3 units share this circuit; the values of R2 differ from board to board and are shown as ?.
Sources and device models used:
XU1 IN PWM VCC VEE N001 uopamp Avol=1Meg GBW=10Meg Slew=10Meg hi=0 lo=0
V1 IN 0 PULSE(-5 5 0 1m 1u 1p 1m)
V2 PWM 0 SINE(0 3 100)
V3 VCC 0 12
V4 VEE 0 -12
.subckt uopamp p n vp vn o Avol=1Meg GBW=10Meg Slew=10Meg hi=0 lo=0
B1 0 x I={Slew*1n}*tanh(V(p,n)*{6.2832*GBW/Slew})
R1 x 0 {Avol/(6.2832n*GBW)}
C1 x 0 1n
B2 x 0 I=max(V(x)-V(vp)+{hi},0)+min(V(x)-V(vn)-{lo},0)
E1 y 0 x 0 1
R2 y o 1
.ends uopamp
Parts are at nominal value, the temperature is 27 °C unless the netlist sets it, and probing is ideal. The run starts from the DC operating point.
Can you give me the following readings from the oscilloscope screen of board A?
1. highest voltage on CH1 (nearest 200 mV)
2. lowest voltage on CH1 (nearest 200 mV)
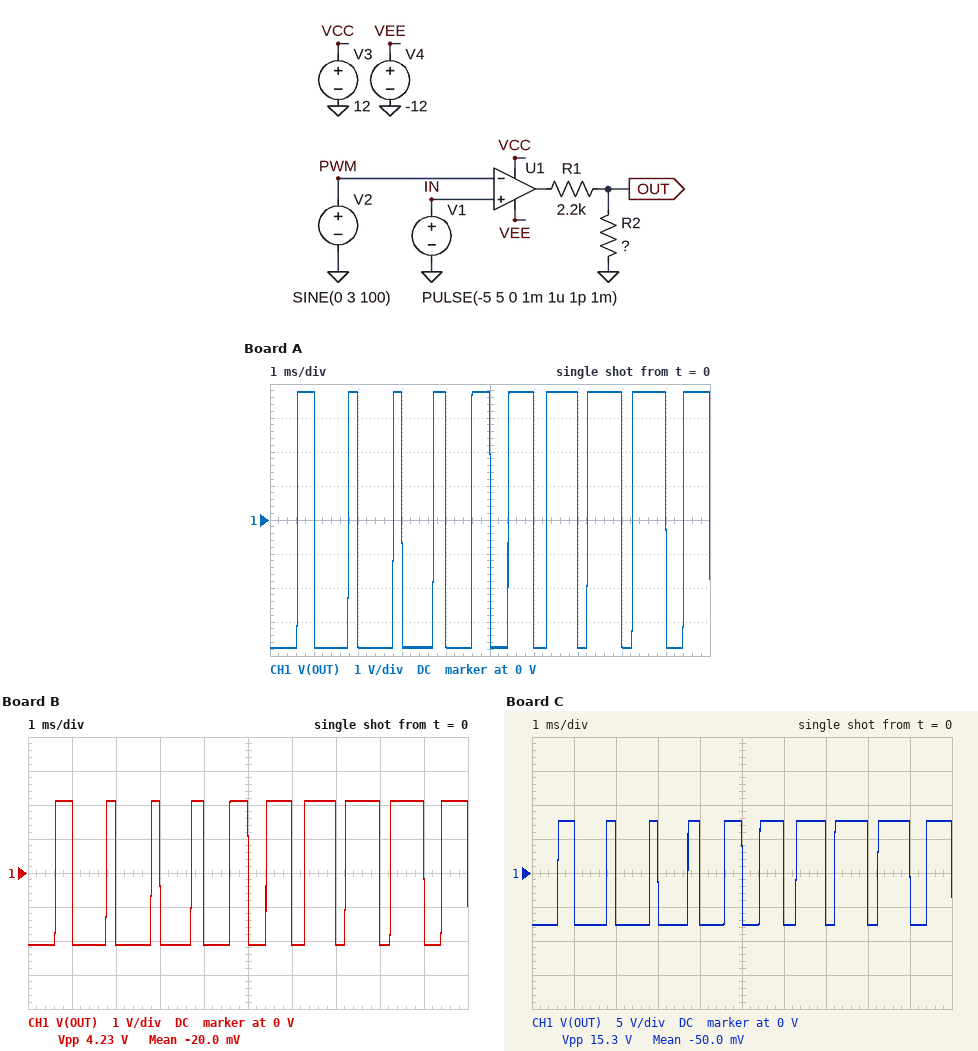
3.8 V
-3.8 V
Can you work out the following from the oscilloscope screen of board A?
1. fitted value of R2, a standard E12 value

1 kΩ
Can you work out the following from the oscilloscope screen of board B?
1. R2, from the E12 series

470 Ω
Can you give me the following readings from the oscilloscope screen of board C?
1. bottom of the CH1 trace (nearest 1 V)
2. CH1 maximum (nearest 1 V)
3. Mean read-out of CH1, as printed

-8 V
8 V
-50.0 mV
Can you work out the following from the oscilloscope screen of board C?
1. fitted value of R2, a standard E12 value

3.9 kΩ
